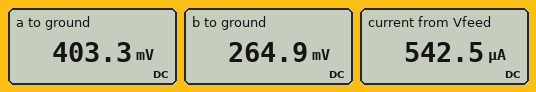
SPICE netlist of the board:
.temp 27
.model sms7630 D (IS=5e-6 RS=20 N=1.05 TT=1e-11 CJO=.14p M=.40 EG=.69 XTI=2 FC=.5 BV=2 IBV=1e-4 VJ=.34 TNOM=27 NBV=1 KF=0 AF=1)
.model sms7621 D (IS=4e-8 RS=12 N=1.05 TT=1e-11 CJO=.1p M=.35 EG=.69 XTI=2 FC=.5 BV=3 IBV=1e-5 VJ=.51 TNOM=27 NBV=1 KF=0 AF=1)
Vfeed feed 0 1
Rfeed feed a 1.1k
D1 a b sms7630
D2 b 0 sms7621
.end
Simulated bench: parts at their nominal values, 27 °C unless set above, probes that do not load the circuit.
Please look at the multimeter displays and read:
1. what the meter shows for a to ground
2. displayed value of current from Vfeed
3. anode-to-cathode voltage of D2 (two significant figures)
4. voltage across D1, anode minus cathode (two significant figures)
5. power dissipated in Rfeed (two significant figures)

403.3 mV
542.5 µA
260 mV
140 mV
320 µW
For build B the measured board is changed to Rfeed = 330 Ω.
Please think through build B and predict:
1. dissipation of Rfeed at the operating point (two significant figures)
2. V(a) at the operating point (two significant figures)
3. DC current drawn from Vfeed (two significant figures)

780 µW
490 mV
1.5 mA
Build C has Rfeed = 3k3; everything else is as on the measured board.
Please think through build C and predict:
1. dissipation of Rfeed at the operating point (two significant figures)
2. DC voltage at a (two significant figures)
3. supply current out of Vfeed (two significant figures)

130 µW
340 mV
200 µA
